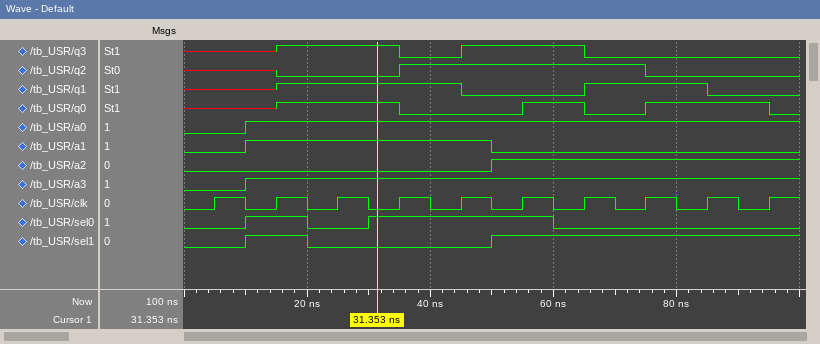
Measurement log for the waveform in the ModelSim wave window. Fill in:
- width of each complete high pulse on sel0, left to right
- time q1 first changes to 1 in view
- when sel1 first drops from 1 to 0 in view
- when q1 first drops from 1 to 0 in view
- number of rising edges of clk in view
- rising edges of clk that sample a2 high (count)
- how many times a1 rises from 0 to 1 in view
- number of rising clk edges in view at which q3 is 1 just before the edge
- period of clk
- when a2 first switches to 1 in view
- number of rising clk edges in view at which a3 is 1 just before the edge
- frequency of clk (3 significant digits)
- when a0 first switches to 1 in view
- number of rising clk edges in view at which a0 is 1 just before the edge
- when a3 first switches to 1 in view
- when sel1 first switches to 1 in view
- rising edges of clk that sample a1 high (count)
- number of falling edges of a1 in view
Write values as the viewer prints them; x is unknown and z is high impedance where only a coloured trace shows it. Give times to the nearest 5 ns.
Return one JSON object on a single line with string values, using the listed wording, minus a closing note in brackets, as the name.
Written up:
{"width of each complete high pulse on sel0, left to right": "10 ns, 30 ns", "time q1 first changes to 1 in view": "15 ns", "when sel1 first drops from 1 to 0 in view": "20 ns", "when q1 first drops from 1 to 0 in view": "45 ns", "number of rising edges of clk in view": "10", "rising edges of clk that sample a2 high": "5", "how many times a1 rises from 0 to 1 in view": "1", "number of rising clk edges in view at which q3 is 1 just before the edge": "4", "period of clk": "10 ns", "when a2 first switches to 1 in view": "50 ns", "number of rising clk edges in view at which a3 is 1 just before the edge": "9", "frequency of clk": "100 MHz", "when a0 first switches to 1 in view": "10 ns", "number of rising clk edges in view at which a0 is 1 just before the edge": "9", "when a3 first switches to 1 in view": "10 ns", "when sel1 first switches to 1 in view": "10 ns", "rising edges of clk that sample a1 high": "4", "number of falling edges of a1 in view": "1"}
